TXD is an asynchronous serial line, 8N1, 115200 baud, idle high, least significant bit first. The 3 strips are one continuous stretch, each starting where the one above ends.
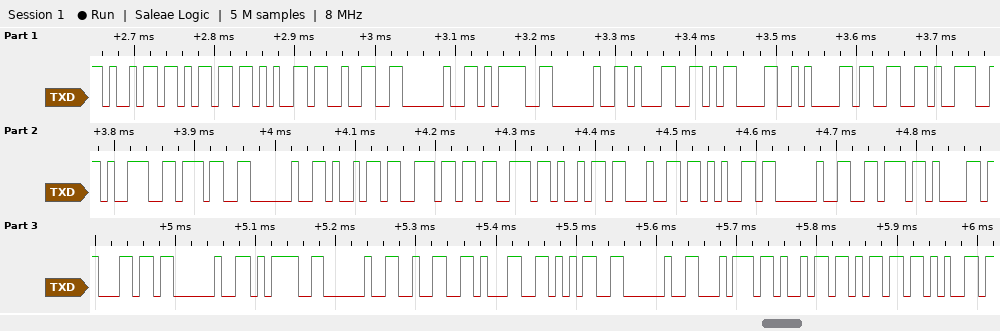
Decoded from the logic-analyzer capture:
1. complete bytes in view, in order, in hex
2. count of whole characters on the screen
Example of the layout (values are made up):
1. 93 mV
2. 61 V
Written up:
1. 0x69 0x6D 0x65 0x32 0x20 0x3D 0x20 0x31 0x0D 0x0A 0x33 0x39 0x39 0x37 0x20 0x69 0x6E 0x73 0x69 0x64 0x65 0x20 0x76 0x61 0x6C 0x20 0x3D 0x20 0x32 0x31 0x35 0x20 0x74 0x69 0x6D 0x65
2. 36
